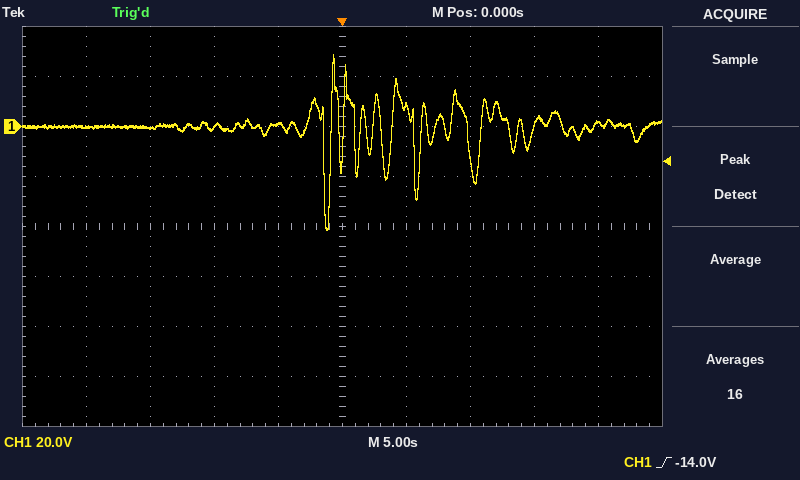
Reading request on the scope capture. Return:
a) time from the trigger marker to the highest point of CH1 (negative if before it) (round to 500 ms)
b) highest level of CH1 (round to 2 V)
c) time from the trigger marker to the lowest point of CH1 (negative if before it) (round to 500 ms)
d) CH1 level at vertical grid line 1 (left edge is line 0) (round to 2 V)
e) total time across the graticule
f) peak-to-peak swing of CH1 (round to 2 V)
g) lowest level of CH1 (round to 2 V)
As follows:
-500 ms
28 V
-1.0 s
0 V
50 s
70 V
-42 V
